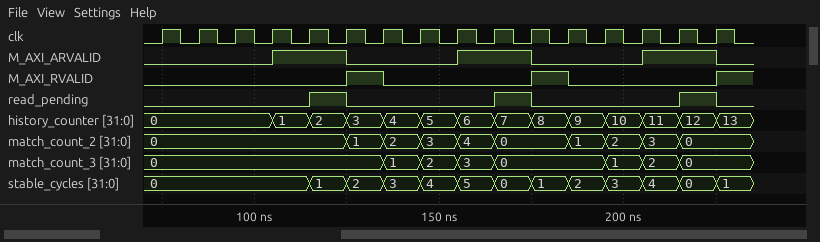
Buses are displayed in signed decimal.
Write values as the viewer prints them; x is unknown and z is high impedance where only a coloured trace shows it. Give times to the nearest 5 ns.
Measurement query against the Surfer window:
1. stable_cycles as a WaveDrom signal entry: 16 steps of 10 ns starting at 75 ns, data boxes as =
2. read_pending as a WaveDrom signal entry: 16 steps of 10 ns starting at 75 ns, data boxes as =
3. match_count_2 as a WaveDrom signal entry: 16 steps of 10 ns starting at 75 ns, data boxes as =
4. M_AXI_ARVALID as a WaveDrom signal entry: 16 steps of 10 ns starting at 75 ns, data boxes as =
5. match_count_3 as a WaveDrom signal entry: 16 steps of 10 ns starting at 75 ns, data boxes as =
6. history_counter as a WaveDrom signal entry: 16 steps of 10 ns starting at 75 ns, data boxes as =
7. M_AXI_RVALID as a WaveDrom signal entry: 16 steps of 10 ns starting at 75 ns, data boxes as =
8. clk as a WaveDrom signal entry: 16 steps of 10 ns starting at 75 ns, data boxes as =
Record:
{name: 'stable_cycles', wave: '=...============', data: '0 1 2 3 4 5 0 1 2 3 4 0 1'}
{name: 'read_pending', wave: '0...10...10...10'}
{name: 'match_count_2', wave: '=....=====.====.', data: '0 1 2 3 4 0 1 2 3 0'}
{name: 'M_AXI_ARVALID', wave: '0..1.0..1.0..1.0'}
{name: 'match_count_3', wave: '=.....====..===.', data: '0 1 2 3 0 1 2 0'}
{name: 'history_counter', wave: '=..=============', data: '0 1 2 3 4 5 6 7 8 9 10 11 12 13'}
{name: 'M_AXI_RVALID', wave: '0....10...10...1'}
{name: 'clk', wave: 'p...............'}
